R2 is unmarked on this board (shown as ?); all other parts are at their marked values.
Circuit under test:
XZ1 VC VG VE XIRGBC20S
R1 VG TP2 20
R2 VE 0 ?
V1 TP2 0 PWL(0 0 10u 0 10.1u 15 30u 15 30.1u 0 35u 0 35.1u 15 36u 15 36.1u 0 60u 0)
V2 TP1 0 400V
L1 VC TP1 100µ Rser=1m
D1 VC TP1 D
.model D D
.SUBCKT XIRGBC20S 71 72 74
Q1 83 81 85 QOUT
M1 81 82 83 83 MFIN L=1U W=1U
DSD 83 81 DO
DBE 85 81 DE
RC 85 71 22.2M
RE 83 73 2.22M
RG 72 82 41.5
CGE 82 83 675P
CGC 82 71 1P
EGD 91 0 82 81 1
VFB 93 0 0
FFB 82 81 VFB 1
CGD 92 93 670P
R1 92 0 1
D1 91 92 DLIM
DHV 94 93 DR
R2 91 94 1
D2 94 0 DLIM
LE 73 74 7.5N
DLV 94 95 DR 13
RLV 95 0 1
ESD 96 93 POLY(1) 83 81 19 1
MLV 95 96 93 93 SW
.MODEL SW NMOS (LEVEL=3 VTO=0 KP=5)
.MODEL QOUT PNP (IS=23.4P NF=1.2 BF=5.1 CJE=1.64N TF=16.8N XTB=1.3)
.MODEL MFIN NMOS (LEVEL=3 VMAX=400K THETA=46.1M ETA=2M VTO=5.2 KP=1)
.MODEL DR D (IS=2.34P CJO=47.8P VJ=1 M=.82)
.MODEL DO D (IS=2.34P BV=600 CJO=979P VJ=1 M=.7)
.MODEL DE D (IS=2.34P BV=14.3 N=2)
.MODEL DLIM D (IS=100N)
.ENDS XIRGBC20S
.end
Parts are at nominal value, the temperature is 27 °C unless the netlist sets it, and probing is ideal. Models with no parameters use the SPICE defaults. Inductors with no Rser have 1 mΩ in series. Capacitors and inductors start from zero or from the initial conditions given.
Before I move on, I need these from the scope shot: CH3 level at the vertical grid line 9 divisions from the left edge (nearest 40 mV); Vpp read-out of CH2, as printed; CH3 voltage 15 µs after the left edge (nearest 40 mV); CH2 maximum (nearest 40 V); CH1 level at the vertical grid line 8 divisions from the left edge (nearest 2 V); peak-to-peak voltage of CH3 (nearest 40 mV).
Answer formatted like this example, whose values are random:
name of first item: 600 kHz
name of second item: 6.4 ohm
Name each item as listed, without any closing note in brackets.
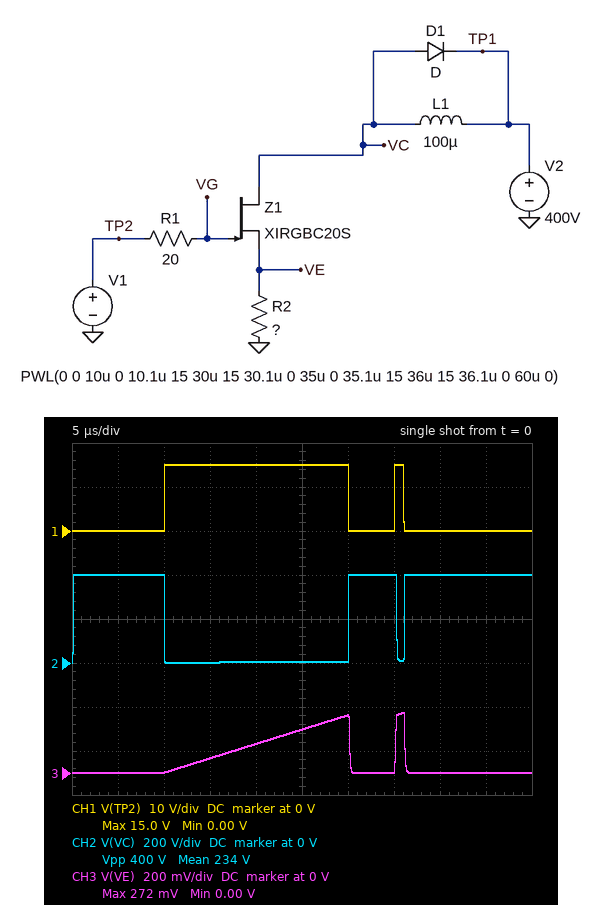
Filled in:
CH3 level at the vertical grid line 9 divisions from the left edge: 0 V
Vpp read-out of CH2, as printed: 400 V
CH3 voltage 15 µs after the left edge: 80 mV
CH2 maximum: 400 V
CH1 level at the vertical grid line 8 divisions from the left edge: 0 V
peak-to-peak voltage of CH3: 280 mV
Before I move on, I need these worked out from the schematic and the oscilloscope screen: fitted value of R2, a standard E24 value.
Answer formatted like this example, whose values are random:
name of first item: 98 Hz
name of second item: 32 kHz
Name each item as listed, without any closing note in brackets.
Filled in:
fitted value of R2, a standard E24 value: 3.3 mΩ
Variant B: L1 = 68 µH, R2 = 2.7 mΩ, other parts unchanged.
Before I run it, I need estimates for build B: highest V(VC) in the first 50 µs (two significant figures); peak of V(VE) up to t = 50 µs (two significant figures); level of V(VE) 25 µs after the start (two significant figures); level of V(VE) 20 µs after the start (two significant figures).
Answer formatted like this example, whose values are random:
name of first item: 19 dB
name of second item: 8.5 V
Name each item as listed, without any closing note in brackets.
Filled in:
highest V(VC) in the first 50 µs: 400 V
peak of V(VE) up to t = 50 µs: 300 mV
level of V(VE) 25 µs after the start: 240 mV
level of V(VE) 20 µs after the start: 160 mV
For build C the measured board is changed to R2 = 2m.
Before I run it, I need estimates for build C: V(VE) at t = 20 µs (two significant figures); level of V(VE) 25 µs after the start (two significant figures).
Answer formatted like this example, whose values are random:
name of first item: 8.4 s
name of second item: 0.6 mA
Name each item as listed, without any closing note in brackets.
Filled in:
V(VE) at t = 20 µs: 80 mV
level of V(VE) 25 µs after the start: 120 mV
